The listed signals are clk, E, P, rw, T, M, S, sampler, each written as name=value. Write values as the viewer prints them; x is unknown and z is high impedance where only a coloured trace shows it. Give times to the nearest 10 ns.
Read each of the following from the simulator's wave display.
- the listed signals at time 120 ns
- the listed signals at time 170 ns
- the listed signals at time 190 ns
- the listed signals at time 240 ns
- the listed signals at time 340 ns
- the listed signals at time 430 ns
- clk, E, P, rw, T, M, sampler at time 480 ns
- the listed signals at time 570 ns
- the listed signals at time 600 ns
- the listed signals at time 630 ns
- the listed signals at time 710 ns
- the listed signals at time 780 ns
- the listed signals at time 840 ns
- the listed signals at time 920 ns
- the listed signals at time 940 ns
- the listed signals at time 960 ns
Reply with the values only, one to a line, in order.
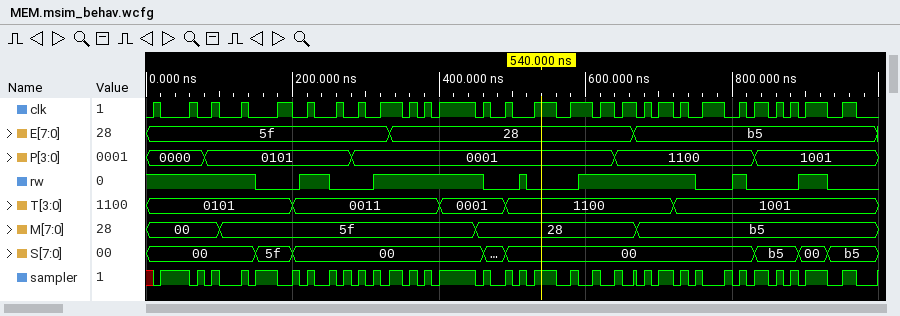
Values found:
clk=0, E=5f, P=0101, rw=1, T=0101, M=5f, S=00, sampler=0
clk=0, E=5f, P=0101, rw=0, T=0101, M=5f, S=5f, sampler=1
clk=1, E=5f, P=0101, rw=0, T=0101, M=5f, S=5f, sampler=0
clk=0, E=5f, P=0101, rw=1, T=0011, M=5f, S=00, sampler=0
clk=1, E=28, P=0001, rw=1, T=0011, M=5f, S=00, sampler=1
clk=1, E=28, P=0001, rw=1, T=0001, M=5f, S=00, sampler=1
clk=0, E=28, P=0001, rw=0, T=0001, M=28, sampler=0
clk=0, E=28, P=0001, rw=0, T=1100, M=28, S=00, sampler=0
clk=1, E=28, P=0001, rw=1, T=1100, M=28, S=00, sampler=0
clk=1, E=28, P=0001, rw=1, T=1100, M=28, S=00, sampler=0
clk=1, E=b5, P=1100, rw=1, T=1100, M=b5, S=00, sampler=1
clk=1, E=b5, P=1100, rw=0, T=1001, M=b5, S=00, sampler=0
clk=1, E=b5, P=1001, rw=0, T=1001, M=b5, S=b5, sampler=1
clk=1, E=b5, P=1001, rw=1, T=1001, M=b5, S=00, sampler=1
clk=0, E=b5, P=1001, rw=0, T=1001, M=b5, S=b5, sampler=0
clk=1, E=b5, P=1001, rw=0, T=1001, M=b5, S=b5, sampler=1
